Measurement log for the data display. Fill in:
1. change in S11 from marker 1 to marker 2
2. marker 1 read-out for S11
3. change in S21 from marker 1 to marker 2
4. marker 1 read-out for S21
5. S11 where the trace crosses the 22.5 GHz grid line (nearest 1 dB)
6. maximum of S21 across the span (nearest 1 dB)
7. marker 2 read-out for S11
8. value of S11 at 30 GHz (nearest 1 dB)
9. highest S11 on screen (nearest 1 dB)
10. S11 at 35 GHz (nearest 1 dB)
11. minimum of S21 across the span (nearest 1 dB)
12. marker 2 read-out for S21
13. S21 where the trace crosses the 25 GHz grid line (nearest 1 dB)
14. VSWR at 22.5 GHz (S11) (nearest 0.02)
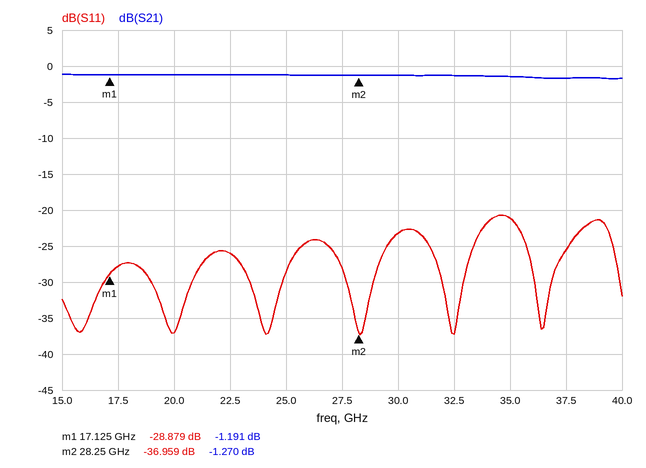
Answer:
-8.080 dB
-28.879 dB
-0.079 dB
-1.191 dB
-26 dB
-1 dB
-36.959 dB
-23 dB
-21 dB
-21 dB
-2 dB
-1.270 dB
-1 dB
1.10
